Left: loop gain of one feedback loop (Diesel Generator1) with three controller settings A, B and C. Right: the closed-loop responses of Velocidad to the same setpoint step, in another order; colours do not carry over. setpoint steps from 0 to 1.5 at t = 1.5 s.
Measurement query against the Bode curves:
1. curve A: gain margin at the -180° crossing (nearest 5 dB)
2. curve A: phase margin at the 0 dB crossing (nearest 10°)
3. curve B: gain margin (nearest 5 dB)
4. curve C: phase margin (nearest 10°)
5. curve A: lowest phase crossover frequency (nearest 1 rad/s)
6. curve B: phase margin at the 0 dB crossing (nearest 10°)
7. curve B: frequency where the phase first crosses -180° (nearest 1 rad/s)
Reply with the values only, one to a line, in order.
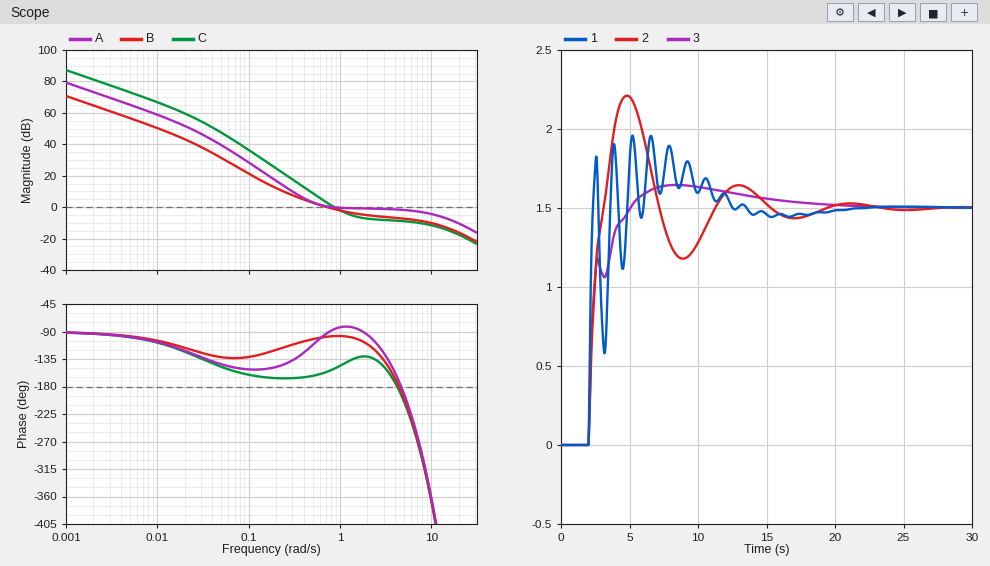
0 dB
90°
5 dB
30°
5 rad/s
80°
4 rad/s
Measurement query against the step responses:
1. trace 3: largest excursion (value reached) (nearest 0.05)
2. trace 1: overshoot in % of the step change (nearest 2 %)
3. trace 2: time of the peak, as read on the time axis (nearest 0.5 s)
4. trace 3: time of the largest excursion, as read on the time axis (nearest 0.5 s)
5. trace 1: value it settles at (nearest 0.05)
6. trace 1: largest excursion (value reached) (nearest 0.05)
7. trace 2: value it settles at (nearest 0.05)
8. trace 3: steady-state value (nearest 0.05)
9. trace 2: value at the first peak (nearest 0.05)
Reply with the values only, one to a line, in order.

1.65
30 %
5.0 s
8.5 s
1.50
1.95
1.50
1.50
2.20
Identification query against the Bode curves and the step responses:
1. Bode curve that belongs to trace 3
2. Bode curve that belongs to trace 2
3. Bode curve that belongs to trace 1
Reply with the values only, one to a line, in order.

B
C
A
